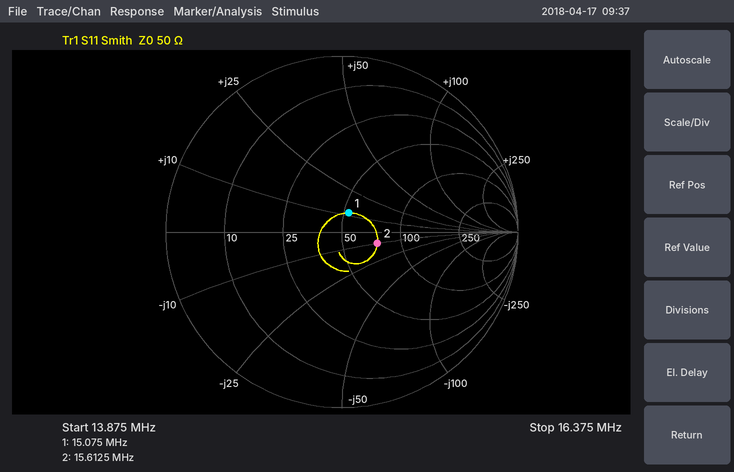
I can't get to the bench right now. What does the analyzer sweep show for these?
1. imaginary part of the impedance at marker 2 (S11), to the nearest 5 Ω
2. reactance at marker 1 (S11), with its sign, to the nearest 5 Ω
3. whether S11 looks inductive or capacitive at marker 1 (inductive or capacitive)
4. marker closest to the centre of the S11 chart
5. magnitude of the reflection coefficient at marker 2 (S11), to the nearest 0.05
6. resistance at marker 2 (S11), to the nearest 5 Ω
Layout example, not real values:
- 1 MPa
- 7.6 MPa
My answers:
- -10 Ω
- +10 Ω
- inductive
- marker 1
- 0.20
- 75 Ω
